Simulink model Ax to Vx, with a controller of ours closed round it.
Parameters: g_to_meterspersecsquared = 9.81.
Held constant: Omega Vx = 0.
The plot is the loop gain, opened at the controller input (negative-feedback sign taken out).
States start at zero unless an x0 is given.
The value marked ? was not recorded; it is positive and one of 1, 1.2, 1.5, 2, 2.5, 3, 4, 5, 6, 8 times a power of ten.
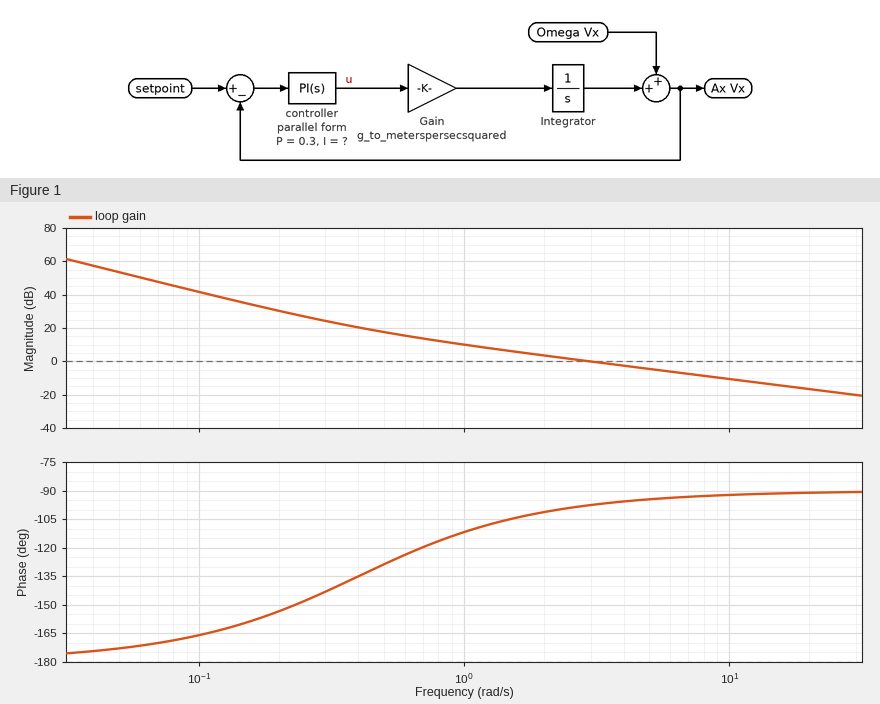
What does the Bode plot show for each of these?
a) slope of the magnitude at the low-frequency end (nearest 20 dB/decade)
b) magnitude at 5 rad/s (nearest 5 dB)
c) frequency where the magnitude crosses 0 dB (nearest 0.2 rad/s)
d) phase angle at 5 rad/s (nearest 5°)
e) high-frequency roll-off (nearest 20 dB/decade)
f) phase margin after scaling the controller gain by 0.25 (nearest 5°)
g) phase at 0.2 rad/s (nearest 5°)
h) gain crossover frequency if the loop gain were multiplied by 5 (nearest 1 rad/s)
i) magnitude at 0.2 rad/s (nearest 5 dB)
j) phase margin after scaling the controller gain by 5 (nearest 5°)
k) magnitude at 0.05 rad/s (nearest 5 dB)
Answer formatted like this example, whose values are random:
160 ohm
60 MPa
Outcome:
-40 dB/decade
-5 dB
3.0 rad/s
-95°
-20 dB/decade
65°
-155°
15 rad/s
30 dB
90°
55 dB
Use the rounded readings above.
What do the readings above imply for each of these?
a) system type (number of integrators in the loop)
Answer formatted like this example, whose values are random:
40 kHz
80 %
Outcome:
2
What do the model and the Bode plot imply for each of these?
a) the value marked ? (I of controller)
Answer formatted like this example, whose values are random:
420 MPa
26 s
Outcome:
0.12
